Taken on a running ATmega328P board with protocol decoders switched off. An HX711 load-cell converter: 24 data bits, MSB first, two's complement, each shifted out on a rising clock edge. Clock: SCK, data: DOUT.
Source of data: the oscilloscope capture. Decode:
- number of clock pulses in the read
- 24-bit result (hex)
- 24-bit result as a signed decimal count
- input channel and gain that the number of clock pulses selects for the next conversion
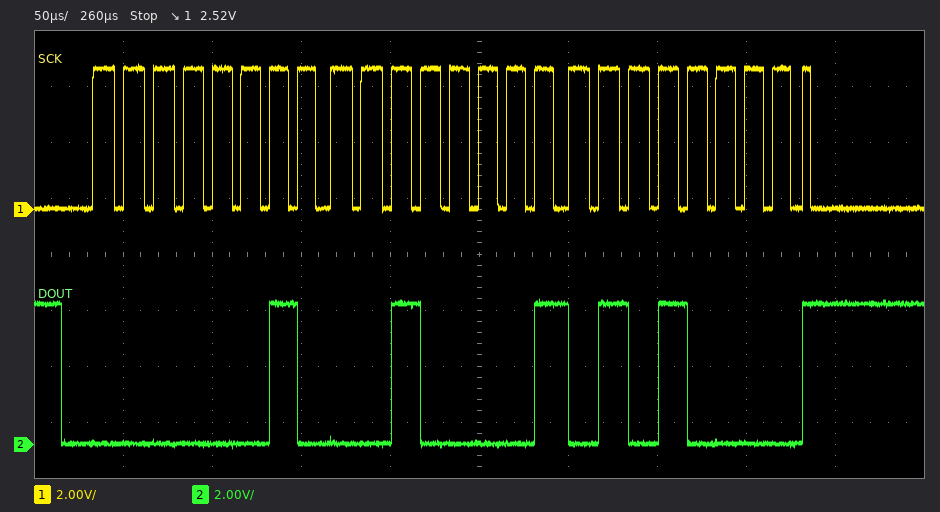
25
0x022150
139600
channel A, gain 128
